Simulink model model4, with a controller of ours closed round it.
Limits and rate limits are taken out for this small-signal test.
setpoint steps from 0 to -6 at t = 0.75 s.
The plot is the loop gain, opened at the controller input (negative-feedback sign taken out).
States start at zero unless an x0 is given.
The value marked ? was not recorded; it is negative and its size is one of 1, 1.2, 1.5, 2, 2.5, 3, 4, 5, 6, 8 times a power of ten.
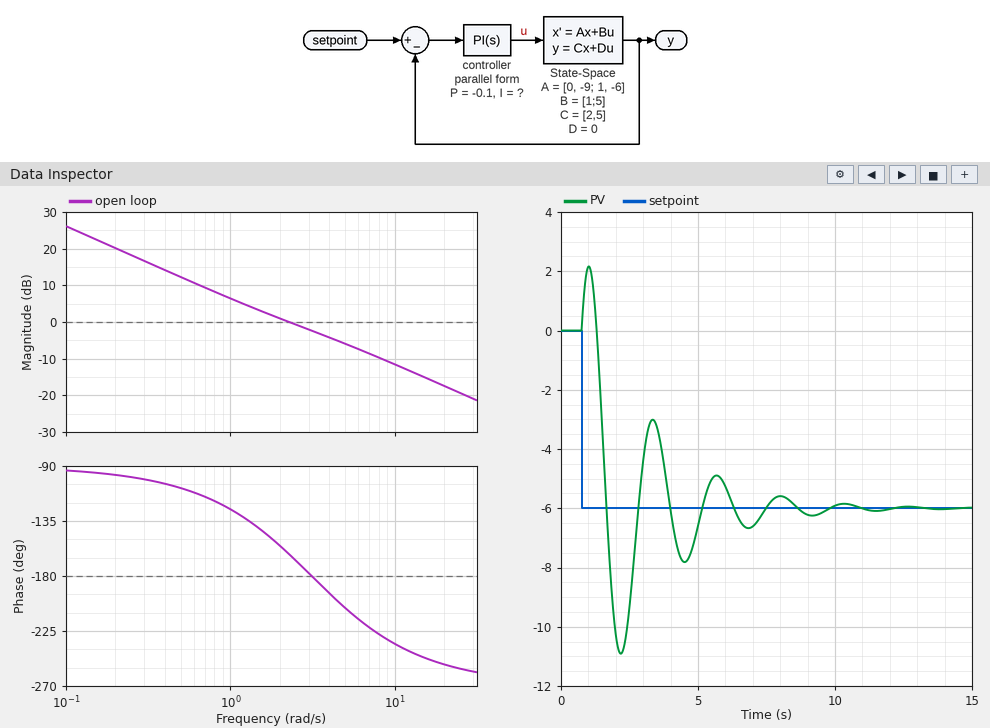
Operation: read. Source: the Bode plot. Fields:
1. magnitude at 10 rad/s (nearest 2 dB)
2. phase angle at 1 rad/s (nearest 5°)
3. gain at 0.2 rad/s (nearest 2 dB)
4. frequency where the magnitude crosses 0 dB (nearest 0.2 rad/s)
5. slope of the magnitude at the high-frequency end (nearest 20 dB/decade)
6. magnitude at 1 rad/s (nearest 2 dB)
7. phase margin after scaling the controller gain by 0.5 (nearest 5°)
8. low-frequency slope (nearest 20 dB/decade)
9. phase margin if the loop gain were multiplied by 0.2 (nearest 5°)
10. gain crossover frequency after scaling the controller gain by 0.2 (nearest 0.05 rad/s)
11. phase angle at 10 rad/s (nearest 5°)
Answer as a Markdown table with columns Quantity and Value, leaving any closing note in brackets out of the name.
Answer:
| Quantity | Value |
|---|---|
| magnitude at 10 rad/s | -12 dB |
| phase angle at 1 rad/s | -125° |
| gain at 0.2 rad/s | 20 dB |
| frequency where the magnitude crosses 0 dB | 2.2 rad/s |
| slope of the magnitude at the high-frequency end | -20 dB/decade |
| magnitude at 1 rad/s | 6 dB |
| phase margin after scaling the controller gain by 0.5 | 55° |
| low-frequency slope | -20 dB/decade |
| phase margin if the loop gain were multiplied by 0.2 | 75° |
| gain crossover frequency after scaling the controller gain by 0.2 | 0.40 rad/s |
| phase angle at 10 rad/s | -235° |
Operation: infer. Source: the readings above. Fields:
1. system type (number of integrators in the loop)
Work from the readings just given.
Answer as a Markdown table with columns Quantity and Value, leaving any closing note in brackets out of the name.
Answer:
| Quantity | Value |
|---|---|
| system type | 1 |
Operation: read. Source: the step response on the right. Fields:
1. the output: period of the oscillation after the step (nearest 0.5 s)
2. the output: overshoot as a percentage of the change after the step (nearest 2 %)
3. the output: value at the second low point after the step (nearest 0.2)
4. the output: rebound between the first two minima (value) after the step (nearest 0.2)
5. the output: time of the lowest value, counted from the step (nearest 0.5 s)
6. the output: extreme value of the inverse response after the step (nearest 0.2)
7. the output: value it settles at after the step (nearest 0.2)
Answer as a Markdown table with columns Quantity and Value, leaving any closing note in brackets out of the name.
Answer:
| Quantity | Value |
|---|---|
| the output: period of the oscillation after the step | 2.5 s |
| the output: overshoot as a percentage of the change after the step | 82 % |
| the output: value at the second low point after the step | -7.8 |
| the output: rebound between the first two minima (value) after the step | -3.0 |
| the output: time of the lowest value, counted from the step | 1.5 s |
| the output: extreme value of the inverse response after the step | 2.2 |
| the output: value it settles at after the step | -6.0 |
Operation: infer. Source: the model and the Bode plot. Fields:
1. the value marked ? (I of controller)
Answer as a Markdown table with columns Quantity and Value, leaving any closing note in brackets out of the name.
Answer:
| Quantity | Value |
|---|---|
| the value marked ? | -0.25 |
